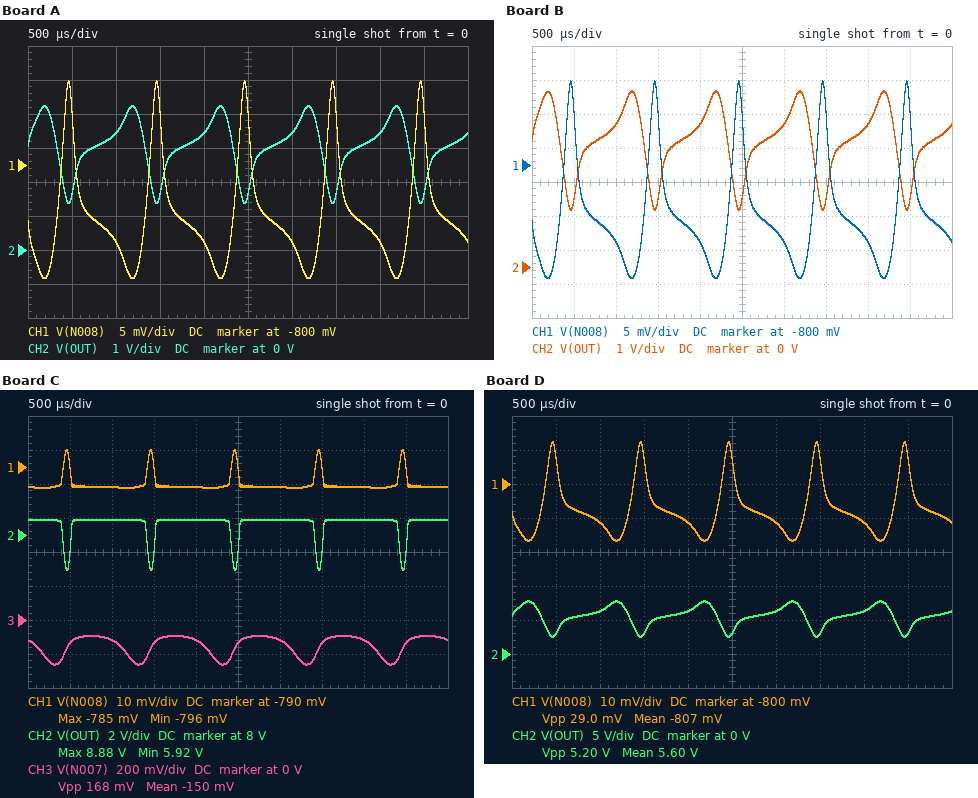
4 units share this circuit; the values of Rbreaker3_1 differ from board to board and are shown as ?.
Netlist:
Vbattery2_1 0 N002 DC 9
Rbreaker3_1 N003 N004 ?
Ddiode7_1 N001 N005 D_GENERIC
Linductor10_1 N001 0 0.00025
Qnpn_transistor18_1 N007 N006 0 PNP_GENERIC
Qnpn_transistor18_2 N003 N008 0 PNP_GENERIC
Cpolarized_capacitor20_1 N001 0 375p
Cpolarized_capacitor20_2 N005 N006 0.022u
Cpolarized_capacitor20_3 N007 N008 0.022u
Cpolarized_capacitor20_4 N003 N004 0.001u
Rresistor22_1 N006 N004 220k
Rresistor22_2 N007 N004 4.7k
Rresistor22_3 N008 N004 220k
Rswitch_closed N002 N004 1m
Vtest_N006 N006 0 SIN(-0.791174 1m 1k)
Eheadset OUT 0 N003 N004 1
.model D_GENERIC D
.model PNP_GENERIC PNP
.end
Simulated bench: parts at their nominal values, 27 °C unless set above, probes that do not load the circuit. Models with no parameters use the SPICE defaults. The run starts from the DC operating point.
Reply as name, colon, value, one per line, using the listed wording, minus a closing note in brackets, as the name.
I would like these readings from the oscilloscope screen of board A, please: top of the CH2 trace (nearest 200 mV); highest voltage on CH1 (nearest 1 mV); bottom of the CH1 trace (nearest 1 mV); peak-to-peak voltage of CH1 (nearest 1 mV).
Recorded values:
top of the CH2 trace: 4.2 V
highest voltage on CH1: -788 mV
bottom of the CH1 trace: -817 mV
peak-to-peak voltage of CH1: 29 mV
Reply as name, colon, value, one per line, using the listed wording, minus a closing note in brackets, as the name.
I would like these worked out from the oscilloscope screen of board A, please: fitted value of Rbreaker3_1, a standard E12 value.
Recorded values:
fitted value of Rbreaker3_1, a standard E12 value: 820 Ω
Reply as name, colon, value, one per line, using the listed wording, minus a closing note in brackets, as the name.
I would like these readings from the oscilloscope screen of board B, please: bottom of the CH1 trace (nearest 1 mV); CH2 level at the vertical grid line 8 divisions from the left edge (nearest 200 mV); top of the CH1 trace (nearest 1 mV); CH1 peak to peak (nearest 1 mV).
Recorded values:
bottom of the CH1 trace: -817 mV
CH2 level at the vertical grid line 8 divisions from the left edge: 4.2 V
top of the CH1 trace: -788 mV
CH1 peak to peak: 29 mV
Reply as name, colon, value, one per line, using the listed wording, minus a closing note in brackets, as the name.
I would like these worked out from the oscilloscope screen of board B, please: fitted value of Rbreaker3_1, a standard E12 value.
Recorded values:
fitted value of Rbreaker3_1, a standard E12 value: 1 kΩ
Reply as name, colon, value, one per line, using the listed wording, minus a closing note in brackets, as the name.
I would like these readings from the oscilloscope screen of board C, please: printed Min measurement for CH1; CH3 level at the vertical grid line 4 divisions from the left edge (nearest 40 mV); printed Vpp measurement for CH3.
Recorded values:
printed Min measurement for CH1: -796 mV
CH3 level at the vertical grid line 4 divisions from the left edge: -120 mV
printed Vpp measurement for CH3: 168 mV
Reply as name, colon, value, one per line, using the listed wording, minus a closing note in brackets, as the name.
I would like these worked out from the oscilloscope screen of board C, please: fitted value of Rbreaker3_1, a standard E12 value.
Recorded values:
fitted value of Rbreaker3_1, a standard E12 value: 3.9 kΩ
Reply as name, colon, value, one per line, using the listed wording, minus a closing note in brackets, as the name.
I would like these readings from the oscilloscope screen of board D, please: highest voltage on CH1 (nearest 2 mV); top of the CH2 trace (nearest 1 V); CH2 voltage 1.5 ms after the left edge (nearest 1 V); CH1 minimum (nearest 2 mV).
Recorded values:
highest voltage on CH1: -788 mV
top of the CH2 trace: 8 V
CH2 voltage 1.5 ms after the left edge: 3 V
CH1 minimum: -816 mV
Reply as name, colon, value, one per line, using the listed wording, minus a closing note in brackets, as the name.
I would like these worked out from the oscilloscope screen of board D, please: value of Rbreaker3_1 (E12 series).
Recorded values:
value of Rbreaker3_1: 1.5 kΩ
